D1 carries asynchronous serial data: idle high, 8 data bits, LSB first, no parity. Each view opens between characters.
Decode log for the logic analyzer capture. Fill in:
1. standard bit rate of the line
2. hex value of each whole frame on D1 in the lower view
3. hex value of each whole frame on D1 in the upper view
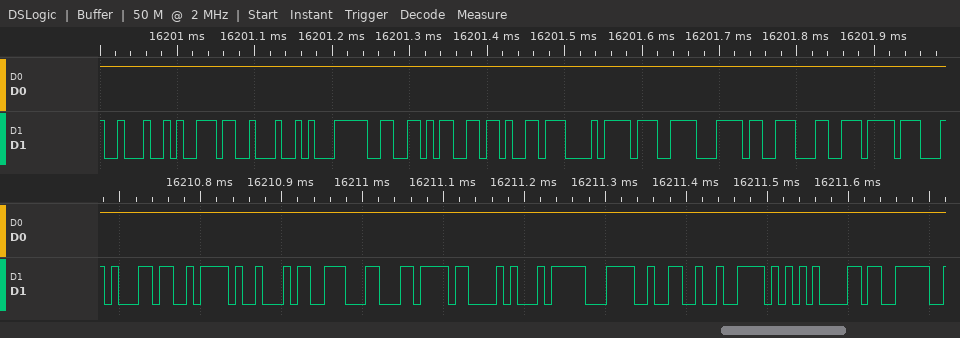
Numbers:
115200 baud
B1, 7A, A2, 8E, EC, 43, F4, 3C, 26, 5E, 85, F3
22, B9, 22, F1, 66, B3, D9, E8, E7, BC, 8E, EE
